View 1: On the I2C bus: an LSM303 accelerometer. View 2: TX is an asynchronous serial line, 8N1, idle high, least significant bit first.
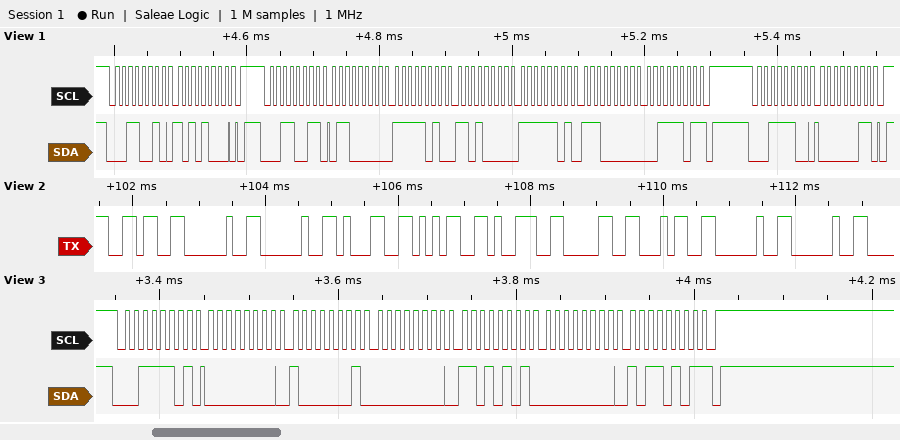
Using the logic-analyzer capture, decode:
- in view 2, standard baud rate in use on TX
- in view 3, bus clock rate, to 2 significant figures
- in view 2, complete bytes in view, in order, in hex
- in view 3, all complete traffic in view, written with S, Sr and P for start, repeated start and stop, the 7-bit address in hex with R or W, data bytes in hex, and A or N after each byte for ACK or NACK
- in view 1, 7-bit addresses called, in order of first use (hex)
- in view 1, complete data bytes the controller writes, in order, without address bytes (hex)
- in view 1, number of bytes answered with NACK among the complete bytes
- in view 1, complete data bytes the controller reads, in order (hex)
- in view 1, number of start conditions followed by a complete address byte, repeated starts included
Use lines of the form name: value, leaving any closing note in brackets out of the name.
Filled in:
in view 2, standard baud rate in use on TX: 9600 baud
in view 3, bus clock rate, to 2 significant figures: 100 kHz
in view 2, complete bytes in view, in order, in hex: 36 20 20 31 35 39 30 34 20 20
in view 3, all complete traffic in view, written with S, Sr and P for start, repeated start and stop, the 7-bit address in hex with R or W, data bytes in hex, and A or N after each byte for ACK or NACK: S 1ER A 00 A 81 A 00 A D5 A 00 A B5 N P
in view 1, 7-bit addresses called, in order of first use: 0x19 0x1E
in view 1, complete data bytes the controller writes, in order, without address bytes: A8 03
in view 1, number of bytes answered with NACK among the complete bytes: 1
in view 1, complete data bytes the controller reads, in order: 60 FA D0 FD E0 3D
in view 1, number of start conditions followed by a complete address byte, repeated starts included: 3
